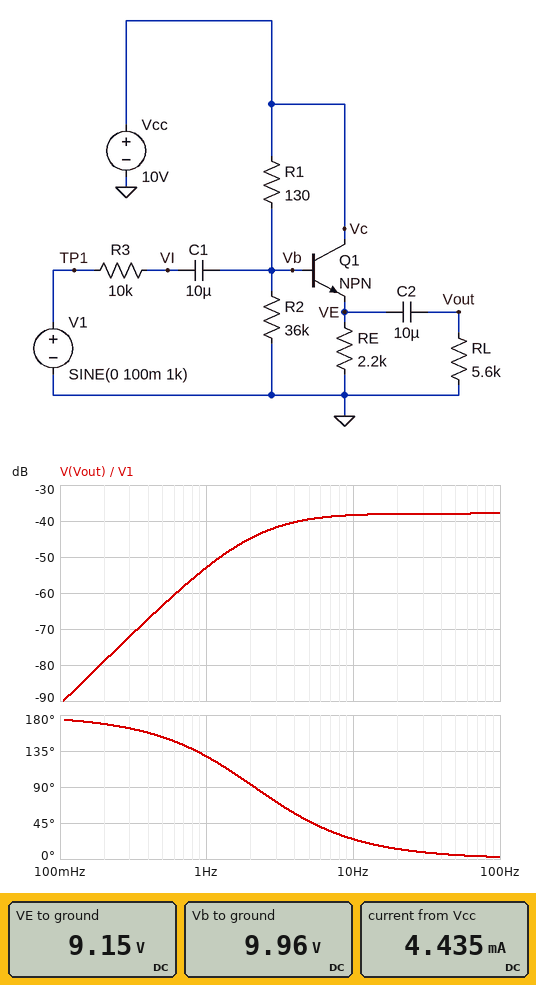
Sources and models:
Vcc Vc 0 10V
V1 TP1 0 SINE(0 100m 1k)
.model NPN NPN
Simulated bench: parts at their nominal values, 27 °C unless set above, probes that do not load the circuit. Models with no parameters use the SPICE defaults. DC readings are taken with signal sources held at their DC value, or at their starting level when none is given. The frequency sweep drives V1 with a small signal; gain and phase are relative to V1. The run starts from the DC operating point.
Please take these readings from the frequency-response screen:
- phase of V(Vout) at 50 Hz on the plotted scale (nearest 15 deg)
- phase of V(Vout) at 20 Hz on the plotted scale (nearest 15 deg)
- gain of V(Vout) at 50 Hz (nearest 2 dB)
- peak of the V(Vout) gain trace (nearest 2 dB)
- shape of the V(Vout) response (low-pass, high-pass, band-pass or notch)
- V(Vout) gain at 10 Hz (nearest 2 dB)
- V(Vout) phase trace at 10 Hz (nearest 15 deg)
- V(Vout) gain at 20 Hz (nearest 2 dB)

0 deg
15 deg
-38 dB
-38 dB
high-pass
-38 dB
30 deg
-38 dB
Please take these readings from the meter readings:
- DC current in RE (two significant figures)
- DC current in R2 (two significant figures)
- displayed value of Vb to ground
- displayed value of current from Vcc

4.2 mA
280 µA
9.96 V
4.435 mA
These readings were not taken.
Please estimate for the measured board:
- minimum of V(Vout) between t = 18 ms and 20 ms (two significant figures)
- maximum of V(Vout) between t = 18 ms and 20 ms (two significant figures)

-1.3 mV
1.3 mV
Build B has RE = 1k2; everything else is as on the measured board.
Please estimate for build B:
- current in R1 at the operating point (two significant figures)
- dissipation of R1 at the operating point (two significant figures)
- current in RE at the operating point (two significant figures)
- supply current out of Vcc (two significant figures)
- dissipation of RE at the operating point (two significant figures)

350 µA
16 µW
7.6 mA
7.9 mA
69 mW
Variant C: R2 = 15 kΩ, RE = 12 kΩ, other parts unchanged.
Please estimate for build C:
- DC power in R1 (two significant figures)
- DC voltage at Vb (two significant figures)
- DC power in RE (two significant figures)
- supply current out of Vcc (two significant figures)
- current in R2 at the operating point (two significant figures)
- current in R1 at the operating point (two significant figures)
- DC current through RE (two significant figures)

58 µW
9.9 V
7.0 mW
1.4 mA
660 µA
670 µA
760 µA
